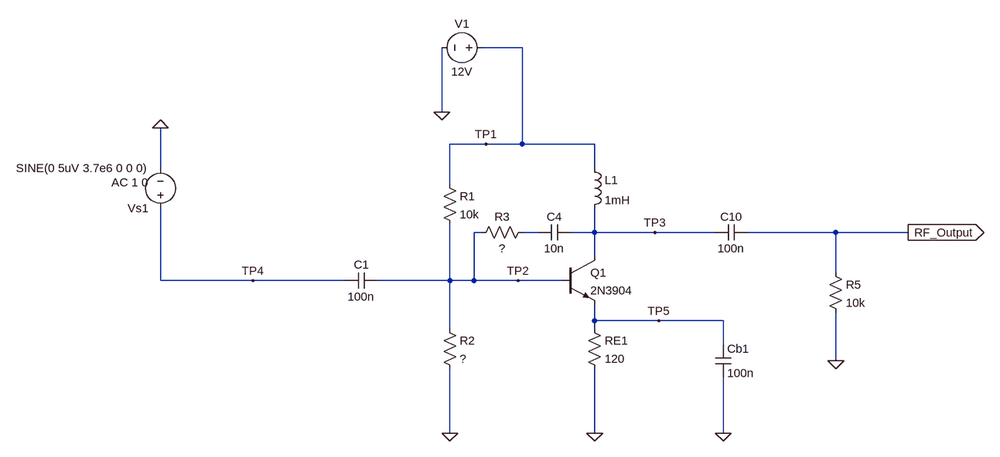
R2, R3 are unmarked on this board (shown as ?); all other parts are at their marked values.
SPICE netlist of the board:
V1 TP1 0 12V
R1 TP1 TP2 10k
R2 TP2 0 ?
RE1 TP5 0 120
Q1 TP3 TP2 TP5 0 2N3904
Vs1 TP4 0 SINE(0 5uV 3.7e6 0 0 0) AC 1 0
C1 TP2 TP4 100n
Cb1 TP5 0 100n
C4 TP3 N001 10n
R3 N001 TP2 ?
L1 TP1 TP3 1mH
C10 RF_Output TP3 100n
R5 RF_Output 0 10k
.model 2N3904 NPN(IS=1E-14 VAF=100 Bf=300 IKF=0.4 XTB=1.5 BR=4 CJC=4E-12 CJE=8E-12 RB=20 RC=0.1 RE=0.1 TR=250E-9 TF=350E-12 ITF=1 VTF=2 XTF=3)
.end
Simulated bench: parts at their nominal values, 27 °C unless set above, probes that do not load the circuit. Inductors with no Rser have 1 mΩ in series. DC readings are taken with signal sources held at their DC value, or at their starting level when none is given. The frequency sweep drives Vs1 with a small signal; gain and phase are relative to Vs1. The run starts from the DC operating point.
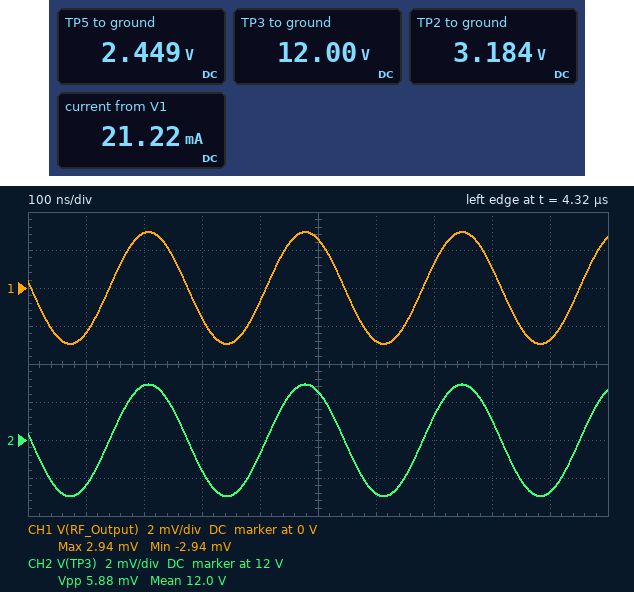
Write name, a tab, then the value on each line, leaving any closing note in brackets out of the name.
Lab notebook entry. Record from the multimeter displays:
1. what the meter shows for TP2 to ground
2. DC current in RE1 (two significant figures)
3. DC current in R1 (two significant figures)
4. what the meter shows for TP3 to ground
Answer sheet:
what the meter shows for TP2 to ground	3.184 V
DC current in RE1	20 mA
DC current in R1	880 µA
what the meter shows for TP3 to ground	12.00 V
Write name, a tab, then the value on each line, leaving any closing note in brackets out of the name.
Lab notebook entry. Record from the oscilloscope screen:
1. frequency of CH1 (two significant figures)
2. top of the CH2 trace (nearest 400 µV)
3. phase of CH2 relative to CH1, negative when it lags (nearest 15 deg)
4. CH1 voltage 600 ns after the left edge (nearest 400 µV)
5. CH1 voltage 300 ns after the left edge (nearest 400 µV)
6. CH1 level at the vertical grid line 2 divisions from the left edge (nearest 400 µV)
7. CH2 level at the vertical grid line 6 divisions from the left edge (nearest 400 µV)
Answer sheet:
frequency of CH1	3.7 MHz
top of the CH2 trace	12.0028 V
phase of CH2 relative to CH1, negative when it lags	0 deg
CH1 voltage 600 ns after the left edge	-2.8 mV
CH1 voltage 300 ns after the left edge	-1.6 mV
CH1 level at the vertical grid line 2 divisions from the left edge	2.8 mV
CH2 level at the vertical grid line 6 divisions from the left edge	11.9972 V
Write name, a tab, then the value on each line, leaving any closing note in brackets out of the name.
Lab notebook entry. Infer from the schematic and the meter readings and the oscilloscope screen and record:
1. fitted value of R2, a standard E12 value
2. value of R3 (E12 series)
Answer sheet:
fitted value of R2, a standard E12 value	3.9 kΩ
value of R3	1.2 kΩ
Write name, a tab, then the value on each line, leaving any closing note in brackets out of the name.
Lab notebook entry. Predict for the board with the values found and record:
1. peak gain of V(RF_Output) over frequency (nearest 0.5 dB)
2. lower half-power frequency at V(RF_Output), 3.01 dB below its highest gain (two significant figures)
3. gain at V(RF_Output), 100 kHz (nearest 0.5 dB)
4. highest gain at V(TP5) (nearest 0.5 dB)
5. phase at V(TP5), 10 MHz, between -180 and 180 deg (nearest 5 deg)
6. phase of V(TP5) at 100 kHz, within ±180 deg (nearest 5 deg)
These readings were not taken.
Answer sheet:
peak gain of V(RF_Output) over frequency	55.5 dB
lower half-power frequency at V(RF_Output), 3.01 dB below its highest gain	1.4 MHz
gain at V(RF_Output), 100 kHz	28.5 dB
highest gain at V(TP5)	-0.5 dB
phase at V(TP5), 10 MHz, between -180 and 180 deg	-140 deg
phase of V(TP5) at 100 kHz, within ±180 deg	-20 deg
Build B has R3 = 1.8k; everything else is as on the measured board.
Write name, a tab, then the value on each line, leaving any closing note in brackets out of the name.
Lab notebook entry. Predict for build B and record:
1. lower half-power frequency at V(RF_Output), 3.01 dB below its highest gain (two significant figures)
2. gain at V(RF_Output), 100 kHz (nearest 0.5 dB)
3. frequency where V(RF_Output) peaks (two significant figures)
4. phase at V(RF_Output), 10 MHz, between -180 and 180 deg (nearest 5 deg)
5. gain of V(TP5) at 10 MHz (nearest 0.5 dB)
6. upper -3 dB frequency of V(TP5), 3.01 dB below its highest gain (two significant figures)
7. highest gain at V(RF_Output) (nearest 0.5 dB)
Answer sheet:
lower half-power frequency at V(RF_Output), 3.01 dB below its highest gain	1.3 MHz
gain at V(RF_Output), 100 kHz	30.0 dB
frequency where V(RF_Output) peaks	2.8 MHz
phase at V(RF_Output), 10 MHz, between -180 and 180 deg	115 deg
gain of V(TP5) at 10 MHz	-28.0 dB
upper -3 dB frequency of V(TP5), 3.01 dB below its highest gain	200 kHz
highest gain at V(RF_Output)	58.0 dB
